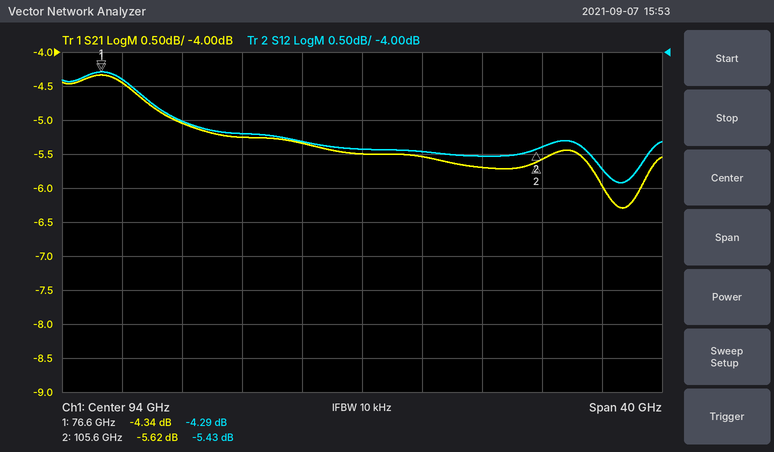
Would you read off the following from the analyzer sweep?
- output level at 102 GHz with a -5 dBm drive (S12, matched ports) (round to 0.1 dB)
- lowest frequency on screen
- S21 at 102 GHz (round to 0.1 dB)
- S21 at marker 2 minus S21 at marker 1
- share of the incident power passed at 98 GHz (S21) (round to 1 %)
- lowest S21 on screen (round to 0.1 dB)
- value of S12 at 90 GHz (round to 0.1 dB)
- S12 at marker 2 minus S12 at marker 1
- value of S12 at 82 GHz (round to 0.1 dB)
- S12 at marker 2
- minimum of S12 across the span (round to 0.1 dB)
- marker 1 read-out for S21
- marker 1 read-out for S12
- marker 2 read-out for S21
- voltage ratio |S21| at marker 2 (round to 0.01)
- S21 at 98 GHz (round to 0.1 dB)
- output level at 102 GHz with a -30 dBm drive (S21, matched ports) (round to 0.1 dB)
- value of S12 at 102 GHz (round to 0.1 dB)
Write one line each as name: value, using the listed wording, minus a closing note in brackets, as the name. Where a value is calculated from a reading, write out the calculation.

output level at 102 GHz with a -5 dBm drive (S12, matched ports): -5 dBm + (-5.5 dB) = -10.5 dBm
lowest frequency on screen: 74 GHz
S21 at 102 GHz: -5.7 dB
S21 at marker 2 minus S21 at marker 1: -5.62 − (-4.34) = -1.28 dB
share of the incident power passed at 98 GHz (S21): 10^(-5.5/10) ≈ 28 %
lowest S21 on screen: -6.3 dB
value of S12 at 90 GHz: -5.3 dB
S12 at marker 2 minus S12 at marker 1: -5.43 − (-4.29) = -1.14 dB
value of S12 at 82 GHz: -5.0 dB
S12 at marker 2: -5.43 dB
minimum of S12 across the span: -5.9 dB
marker 1 read-out for S21: -4.34 dB
marker 1 read-out for S12: -4.29 dB
marker 2 read-out for S21: -5.62 dB
voltage ratio |S21| at marker 2: 10^(-5.62/20) ≈ 0.52
S21 at 98 GHz: -5.5 dB
output level at 102 GHz with a -30 dBm drive (S21, matched ports): -30 dBm + (-5.7 dB) = -35.7 dBm
value of S12 at 102 GHz: -5.5 dB
